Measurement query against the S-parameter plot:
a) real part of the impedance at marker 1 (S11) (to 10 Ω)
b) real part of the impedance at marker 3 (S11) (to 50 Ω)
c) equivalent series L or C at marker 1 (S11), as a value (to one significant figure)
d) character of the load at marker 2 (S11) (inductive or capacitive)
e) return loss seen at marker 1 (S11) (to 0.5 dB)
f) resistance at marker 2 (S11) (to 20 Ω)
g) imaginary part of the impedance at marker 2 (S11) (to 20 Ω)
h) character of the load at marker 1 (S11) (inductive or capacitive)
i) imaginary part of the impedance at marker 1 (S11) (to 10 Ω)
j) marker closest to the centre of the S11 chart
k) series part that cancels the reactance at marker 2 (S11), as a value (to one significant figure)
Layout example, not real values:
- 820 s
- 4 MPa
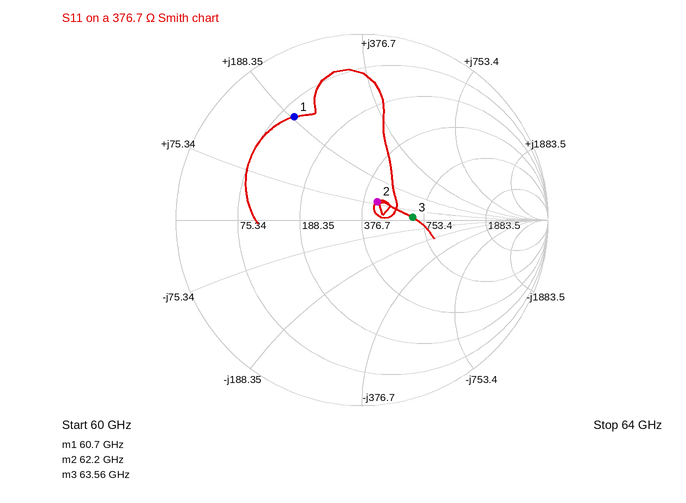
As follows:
- 100 Ω
- 650 Ω
- 500 pH
- inductive
- 3.5 dB
- 440 Ω
- +80 Ω
- inductive
- +190 Ω
- marker 2
- 30 fF
